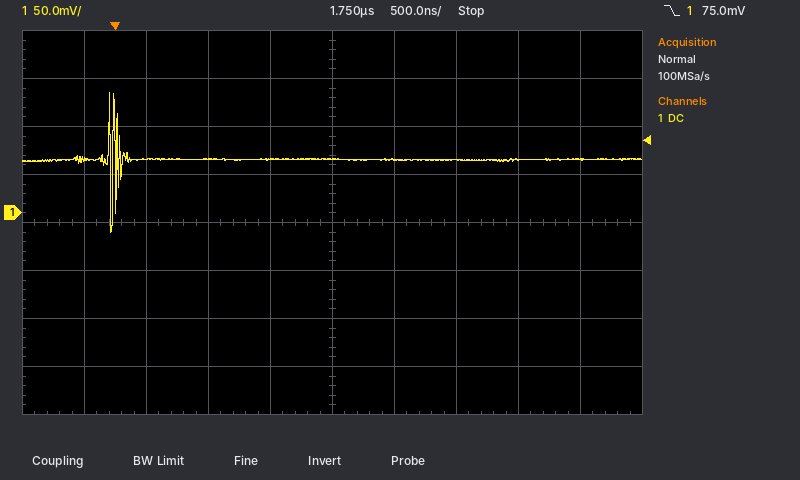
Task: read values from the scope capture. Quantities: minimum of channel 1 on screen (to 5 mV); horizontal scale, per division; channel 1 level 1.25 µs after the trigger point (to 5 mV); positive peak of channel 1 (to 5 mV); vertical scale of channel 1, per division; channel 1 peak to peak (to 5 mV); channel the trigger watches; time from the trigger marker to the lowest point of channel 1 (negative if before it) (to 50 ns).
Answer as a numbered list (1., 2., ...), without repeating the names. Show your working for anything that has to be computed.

1. -20 mV
2. 500 ns
3. 55 mV
4. 125 mV
5. 50 mV
6. 125 mV − (-20 mV) = 145 mV
7. channel 1
8. -50 ns
